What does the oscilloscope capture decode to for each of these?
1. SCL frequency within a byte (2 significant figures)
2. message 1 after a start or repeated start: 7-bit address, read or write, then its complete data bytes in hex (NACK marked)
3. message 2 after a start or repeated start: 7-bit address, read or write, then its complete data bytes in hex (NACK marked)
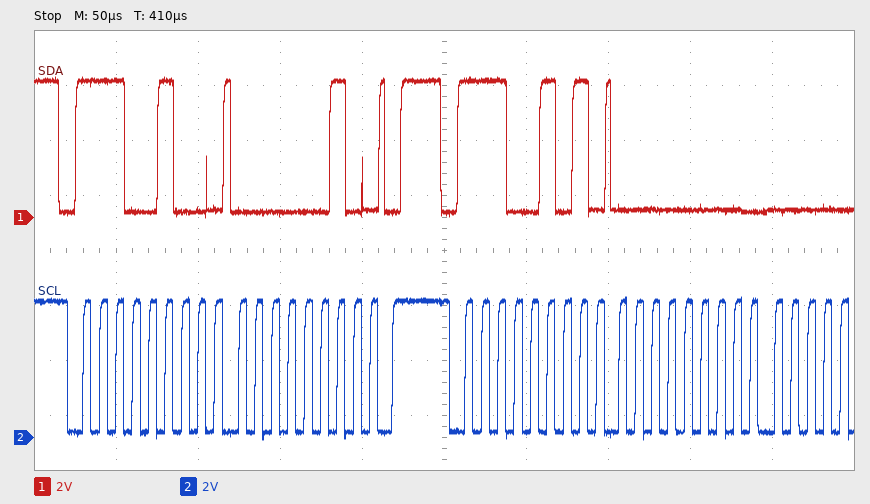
100 kHz
0x72 write: 02
0x72 read: 00
